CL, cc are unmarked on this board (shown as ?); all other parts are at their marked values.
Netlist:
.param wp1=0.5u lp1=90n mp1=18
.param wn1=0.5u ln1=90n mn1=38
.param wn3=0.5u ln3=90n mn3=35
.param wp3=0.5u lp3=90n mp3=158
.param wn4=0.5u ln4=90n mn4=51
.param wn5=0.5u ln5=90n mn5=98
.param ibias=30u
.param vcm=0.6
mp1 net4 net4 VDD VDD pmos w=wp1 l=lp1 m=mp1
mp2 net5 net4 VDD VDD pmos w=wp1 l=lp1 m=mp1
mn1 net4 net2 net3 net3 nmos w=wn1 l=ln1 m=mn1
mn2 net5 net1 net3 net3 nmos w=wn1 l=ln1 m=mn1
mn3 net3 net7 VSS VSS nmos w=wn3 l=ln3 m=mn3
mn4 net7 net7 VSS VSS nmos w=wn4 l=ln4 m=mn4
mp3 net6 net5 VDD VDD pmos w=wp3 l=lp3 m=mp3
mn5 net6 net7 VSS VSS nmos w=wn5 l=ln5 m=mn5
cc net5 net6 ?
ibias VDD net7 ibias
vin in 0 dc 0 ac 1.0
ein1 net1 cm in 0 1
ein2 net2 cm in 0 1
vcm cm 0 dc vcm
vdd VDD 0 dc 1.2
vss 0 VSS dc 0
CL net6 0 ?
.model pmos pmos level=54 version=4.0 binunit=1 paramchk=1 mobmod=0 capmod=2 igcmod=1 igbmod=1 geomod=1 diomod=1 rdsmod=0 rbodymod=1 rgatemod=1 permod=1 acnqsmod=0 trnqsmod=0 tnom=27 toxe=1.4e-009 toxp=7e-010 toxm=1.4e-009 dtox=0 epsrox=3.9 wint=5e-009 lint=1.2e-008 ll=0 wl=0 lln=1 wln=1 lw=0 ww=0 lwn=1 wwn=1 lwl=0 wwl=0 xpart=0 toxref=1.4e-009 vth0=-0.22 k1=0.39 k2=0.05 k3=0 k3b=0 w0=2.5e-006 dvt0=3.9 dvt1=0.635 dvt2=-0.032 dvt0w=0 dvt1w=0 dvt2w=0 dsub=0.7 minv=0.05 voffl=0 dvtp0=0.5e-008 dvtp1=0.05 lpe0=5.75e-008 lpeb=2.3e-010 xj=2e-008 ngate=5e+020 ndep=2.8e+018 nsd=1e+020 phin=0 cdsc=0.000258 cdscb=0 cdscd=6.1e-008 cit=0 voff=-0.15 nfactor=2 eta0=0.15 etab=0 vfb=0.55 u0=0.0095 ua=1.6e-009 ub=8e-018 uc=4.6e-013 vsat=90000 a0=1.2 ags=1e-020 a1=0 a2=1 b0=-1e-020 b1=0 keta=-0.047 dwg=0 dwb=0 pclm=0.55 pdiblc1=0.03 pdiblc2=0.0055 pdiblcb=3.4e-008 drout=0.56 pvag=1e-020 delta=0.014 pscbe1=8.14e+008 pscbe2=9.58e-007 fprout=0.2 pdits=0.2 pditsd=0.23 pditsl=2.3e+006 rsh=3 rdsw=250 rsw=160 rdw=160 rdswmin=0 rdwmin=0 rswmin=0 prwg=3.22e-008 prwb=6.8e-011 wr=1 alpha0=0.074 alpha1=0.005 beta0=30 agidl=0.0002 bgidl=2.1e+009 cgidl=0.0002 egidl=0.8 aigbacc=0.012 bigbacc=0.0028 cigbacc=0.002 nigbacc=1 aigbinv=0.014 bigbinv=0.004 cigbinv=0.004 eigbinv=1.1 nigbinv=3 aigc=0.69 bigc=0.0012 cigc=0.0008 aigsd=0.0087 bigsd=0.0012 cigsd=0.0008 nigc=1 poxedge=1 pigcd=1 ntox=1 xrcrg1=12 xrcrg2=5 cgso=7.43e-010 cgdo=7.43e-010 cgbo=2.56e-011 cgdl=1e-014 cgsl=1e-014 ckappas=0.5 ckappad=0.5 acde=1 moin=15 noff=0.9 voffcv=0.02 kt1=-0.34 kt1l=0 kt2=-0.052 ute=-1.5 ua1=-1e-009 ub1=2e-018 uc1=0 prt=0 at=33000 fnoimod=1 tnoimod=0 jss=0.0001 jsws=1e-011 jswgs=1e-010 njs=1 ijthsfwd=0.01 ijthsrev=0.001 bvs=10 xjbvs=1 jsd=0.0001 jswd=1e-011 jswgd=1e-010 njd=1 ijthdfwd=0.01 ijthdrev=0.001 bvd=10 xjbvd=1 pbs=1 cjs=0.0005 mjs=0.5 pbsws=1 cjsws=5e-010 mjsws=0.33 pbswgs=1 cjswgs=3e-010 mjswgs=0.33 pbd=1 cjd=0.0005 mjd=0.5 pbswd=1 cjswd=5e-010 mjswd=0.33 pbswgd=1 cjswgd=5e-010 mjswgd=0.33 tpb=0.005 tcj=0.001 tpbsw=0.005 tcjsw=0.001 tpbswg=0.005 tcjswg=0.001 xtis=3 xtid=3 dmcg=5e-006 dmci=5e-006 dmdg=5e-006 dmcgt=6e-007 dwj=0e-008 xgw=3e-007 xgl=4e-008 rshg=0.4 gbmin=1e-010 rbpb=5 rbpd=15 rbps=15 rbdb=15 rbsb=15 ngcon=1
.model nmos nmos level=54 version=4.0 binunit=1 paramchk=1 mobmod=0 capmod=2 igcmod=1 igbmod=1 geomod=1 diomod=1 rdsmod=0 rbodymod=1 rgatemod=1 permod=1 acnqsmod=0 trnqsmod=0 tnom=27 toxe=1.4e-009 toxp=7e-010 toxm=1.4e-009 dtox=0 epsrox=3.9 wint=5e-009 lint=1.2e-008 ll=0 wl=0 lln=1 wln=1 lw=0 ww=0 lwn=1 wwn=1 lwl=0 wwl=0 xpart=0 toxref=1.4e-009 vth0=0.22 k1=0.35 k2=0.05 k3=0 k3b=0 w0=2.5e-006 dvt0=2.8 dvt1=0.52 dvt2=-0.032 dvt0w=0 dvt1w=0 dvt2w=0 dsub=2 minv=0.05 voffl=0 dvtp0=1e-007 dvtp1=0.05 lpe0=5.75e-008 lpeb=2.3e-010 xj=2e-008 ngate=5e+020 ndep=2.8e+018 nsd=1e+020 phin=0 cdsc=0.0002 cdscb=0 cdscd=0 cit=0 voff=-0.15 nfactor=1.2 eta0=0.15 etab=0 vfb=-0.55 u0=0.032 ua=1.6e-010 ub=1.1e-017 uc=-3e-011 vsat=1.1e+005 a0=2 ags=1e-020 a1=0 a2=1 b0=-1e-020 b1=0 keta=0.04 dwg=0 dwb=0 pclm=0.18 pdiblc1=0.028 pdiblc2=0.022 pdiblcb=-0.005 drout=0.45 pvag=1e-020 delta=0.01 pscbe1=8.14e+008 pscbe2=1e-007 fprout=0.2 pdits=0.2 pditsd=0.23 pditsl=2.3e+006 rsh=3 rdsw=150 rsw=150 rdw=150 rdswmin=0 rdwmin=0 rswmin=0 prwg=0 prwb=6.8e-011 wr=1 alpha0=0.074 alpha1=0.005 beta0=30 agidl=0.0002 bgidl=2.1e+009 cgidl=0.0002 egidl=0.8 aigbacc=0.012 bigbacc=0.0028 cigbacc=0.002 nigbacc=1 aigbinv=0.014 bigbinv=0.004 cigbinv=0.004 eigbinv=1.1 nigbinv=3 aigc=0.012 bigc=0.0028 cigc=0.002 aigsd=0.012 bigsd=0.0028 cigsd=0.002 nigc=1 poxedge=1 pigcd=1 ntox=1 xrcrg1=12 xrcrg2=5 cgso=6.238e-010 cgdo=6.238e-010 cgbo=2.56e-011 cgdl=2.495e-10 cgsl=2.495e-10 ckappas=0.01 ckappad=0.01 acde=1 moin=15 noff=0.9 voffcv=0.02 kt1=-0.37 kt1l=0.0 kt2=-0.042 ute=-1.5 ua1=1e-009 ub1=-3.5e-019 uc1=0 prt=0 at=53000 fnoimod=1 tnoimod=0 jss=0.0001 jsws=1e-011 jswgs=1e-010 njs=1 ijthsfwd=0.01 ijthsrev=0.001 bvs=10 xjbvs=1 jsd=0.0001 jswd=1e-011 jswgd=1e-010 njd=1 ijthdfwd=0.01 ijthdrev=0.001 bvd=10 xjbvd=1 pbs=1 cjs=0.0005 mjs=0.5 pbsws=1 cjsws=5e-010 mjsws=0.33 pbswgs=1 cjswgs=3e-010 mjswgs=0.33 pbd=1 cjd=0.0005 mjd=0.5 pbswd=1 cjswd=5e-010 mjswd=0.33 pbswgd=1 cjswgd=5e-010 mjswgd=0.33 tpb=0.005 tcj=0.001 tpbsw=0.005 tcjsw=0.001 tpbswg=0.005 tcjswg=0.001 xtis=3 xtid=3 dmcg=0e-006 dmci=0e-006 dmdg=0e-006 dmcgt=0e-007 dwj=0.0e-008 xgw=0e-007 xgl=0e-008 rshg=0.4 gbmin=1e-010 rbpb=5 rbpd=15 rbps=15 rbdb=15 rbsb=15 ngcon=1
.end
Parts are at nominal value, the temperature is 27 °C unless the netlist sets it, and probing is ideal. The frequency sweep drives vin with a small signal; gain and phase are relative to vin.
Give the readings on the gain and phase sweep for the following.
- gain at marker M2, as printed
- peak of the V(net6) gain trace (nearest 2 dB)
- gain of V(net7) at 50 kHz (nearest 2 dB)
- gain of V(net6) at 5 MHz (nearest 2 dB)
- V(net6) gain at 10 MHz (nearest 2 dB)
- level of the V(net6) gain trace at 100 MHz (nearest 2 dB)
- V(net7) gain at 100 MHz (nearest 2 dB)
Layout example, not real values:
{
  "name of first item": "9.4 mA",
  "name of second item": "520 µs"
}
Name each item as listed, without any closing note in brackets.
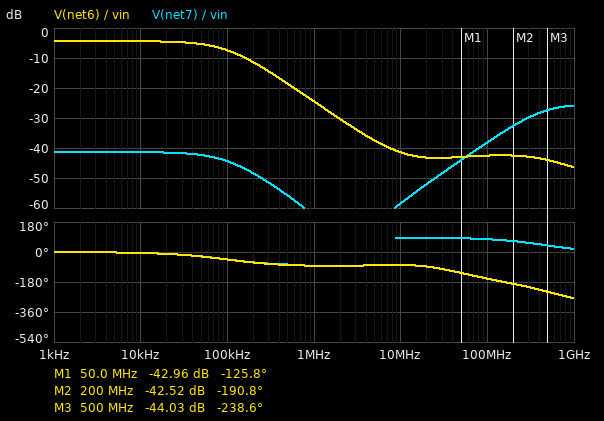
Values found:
{
  "gain at marker M2, as printed": "-42.52 dB",
  "peak of the V(net6) gain trace": "-4 dB",
  "gain of V(net7) at 50 kHz": "-42 dB",
  "gain of V(net6) at 5 MHz": "-38 dB",
  "V(net6) gain at 10 MHz": "-42 dB",
  "level of the V(net6) gain trace at 100 MHz": "-42 dB",
  "V(net7) gain at 100 MHz": "-38 dB"
}
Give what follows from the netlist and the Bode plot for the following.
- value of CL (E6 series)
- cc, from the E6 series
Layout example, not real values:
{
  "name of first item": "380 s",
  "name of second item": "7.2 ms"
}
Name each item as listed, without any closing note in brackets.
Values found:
{
  "value of CL": "4.7 pF",
  "cc, from the E6 series": "1 pF"
}
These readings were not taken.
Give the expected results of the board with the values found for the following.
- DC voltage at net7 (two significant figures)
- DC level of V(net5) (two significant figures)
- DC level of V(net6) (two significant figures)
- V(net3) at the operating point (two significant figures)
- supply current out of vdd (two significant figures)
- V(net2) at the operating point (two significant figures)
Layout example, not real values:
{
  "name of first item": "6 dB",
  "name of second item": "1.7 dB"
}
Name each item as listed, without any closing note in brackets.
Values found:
{
  "DC voltage at net7": "300 mV",
  "DC level of V(net5)": "870 mV",
  "DC level of V(net6)": "940 mV",
  "V(net3) at the operating point": "340 mV",
  "supply current out of vdd": "140 µA",
  "V(net2) at the operating point": "600 mV"
}
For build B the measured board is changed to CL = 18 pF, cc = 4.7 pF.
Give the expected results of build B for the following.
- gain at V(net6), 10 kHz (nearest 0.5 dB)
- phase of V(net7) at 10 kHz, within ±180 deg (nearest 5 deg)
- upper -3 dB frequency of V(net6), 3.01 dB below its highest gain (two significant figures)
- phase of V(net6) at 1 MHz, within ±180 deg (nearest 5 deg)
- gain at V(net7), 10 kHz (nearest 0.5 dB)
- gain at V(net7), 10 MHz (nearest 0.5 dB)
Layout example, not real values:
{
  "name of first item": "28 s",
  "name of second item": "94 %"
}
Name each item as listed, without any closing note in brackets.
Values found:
{
  "gain at V(net6), 10 kHz": "-5.0 dB",
  "phase of V(net7) at 10 kHz, within ±180 deg": "-25 deg",
  "upper -3 dB frequency of V(net6), 3.01 dB below its highest gain": "23 kHz",
  "phase of V(net6) at 1 MHz, within ±180 deg": "-90 deg",
  "gain at V(net7), 10 kHz": "-42.0 dB",
  "gain at V(net7), 10 MHz": "-58.0 dB"
}
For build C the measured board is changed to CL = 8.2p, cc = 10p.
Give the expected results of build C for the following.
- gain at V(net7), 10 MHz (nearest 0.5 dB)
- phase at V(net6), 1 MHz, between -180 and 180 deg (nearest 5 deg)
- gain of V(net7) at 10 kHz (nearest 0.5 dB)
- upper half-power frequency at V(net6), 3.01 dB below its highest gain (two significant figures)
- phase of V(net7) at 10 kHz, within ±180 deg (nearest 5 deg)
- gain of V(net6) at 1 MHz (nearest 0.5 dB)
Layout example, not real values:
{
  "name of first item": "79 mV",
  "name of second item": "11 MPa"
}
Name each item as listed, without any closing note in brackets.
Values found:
{
  "gain at V(net7), 10 MHz": "-58.0 dB",
  "phase at V(net6), 1 MHz, between -180 and 180 deg": "-90 deg",
  "gain of V(net7) at 10 kHz": "-44.0 dB",
  "upper half-power frequency at V(net6), 3.01 dB below its highest gain": "11 kHz",
  "phase of V(net7) at 10 kHz, within ±180 deg": "-40 deg",
  "gain of V(net6) at 1 MHz": "-43.5 dB"
}
